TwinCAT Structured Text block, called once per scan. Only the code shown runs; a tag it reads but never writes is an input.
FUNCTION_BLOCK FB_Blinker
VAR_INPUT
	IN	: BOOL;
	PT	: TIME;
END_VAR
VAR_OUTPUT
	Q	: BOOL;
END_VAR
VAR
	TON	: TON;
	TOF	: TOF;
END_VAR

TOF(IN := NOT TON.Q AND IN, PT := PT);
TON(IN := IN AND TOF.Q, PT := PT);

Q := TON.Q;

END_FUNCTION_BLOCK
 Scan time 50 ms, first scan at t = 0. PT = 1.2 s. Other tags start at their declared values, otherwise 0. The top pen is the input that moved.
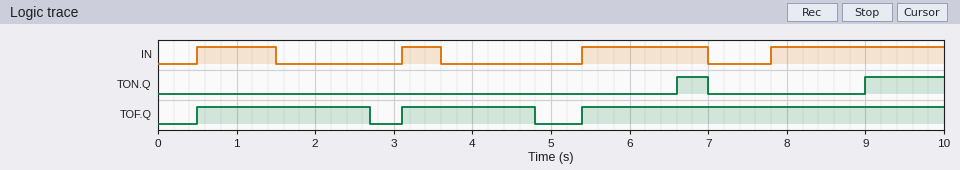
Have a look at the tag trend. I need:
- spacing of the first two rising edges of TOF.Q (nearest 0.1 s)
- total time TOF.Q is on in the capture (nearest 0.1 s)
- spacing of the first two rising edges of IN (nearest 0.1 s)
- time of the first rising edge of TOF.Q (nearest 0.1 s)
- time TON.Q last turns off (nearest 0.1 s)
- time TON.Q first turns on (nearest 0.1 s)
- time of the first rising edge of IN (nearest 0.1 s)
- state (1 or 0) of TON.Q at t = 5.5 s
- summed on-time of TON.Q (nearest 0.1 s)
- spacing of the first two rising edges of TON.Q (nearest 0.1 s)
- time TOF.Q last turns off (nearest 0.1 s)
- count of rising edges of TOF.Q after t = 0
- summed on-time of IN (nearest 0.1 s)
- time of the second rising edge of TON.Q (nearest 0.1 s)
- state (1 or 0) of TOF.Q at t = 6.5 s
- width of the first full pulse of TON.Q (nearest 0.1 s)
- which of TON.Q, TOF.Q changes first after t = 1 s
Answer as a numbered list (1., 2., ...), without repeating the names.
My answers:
1. 2.6 s
2. 8.5 s
3. 2.6 s
4. 0.5 s
5. 7.0 s
6. 6.6 s
7. 0.5 s
8. 0
9. 1.4 s
10. 2.4 s
11. 4.8 s
12. 3
13. 5.3 s
14. 9.0 s
15. 1
16. 0.4 s
17. TOF.Q
